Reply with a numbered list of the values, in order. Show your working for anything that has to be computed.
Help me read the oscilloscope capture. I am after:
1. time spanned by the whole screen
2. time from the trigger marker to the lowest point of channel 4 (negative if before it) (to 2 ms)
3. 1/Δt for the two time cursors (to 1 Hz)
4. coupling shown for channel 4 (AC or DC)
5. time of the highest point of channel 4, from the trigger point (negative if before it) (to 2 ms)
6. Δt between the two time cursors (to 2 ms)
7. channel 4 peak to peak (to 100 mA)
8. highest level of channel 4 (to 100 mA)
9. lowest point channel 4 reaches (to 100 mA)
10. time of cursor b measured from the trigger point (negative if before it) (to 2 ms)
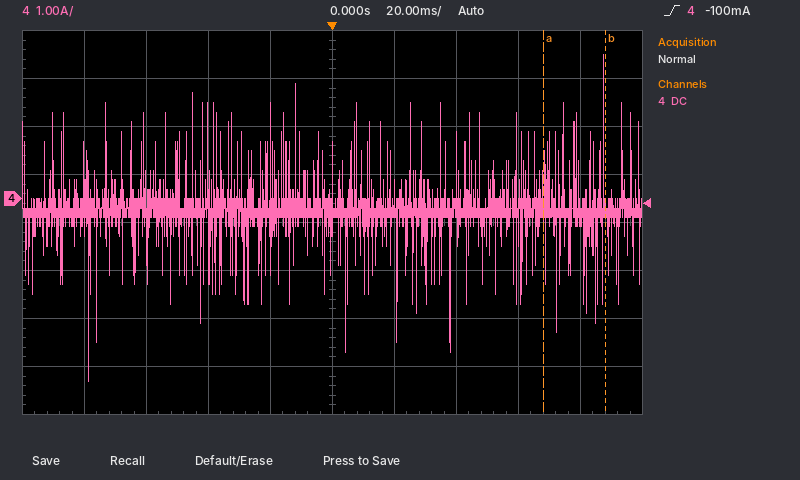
1. 200 ms
2. -78 ms
3. 1 / 20 ms ≈ 50 Hz
4. DC
5. +88 ms
6. 20 ms
7. 3.0 A − (-3.8 A) = 6.8 A
8. 3.0 A
9. -3.8 A
10. +88 ms
